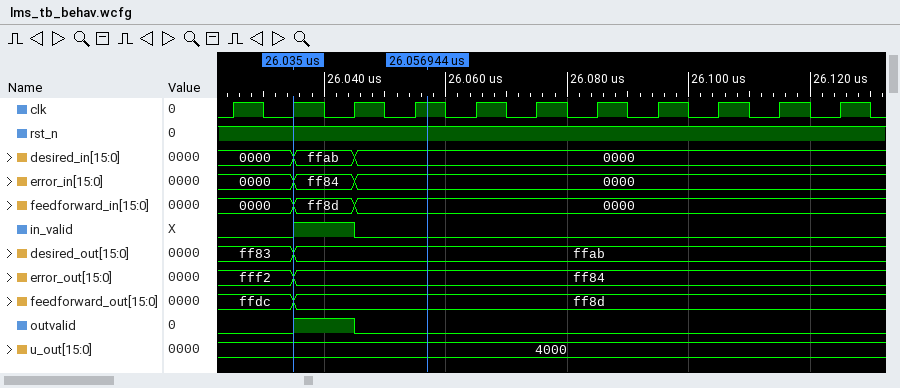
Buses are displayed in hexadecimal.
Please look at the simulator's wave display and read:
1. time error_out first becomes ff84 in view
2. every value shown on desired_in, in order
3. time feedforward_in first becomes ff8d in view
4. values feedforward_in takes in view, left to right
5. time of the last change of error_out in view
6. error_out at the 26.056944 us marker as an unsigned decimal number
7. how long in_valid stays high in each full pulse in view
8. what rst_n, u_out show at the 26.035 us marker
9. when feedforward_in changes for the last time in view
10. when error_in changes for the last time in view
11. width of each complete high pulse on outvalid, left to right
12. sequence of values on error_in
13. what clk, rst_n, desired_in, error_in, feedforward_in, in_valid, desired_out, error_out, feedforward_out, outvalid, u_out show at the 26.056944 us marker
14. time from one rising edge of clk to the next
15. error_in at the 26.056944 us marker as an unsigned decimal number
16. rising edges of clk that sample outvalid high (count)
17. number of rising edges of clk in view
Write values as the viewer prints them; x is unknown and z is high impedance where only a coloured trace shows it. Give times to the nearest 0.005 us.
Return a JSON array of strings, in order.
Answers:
["26.035 us", "0000, ffab, 0000", "26.035 us", "0000, ff8d, 0000", "26.035 us", "65412", "0.01 us", "rst_n=1, u_out=4000", "26.045 us", "26.045 us", "0.01 us", "0000, ff84, 0000", "clk=1, rst_n=1, desired_in=0000, error_in=0000, feedforward_in=0000, in_valid=0, desired_out=ffab, error_out=ff84, feedforward_out=ff8d, outvalid=0, u_out=4000", "0.01 us", "0", "1", "11"]
